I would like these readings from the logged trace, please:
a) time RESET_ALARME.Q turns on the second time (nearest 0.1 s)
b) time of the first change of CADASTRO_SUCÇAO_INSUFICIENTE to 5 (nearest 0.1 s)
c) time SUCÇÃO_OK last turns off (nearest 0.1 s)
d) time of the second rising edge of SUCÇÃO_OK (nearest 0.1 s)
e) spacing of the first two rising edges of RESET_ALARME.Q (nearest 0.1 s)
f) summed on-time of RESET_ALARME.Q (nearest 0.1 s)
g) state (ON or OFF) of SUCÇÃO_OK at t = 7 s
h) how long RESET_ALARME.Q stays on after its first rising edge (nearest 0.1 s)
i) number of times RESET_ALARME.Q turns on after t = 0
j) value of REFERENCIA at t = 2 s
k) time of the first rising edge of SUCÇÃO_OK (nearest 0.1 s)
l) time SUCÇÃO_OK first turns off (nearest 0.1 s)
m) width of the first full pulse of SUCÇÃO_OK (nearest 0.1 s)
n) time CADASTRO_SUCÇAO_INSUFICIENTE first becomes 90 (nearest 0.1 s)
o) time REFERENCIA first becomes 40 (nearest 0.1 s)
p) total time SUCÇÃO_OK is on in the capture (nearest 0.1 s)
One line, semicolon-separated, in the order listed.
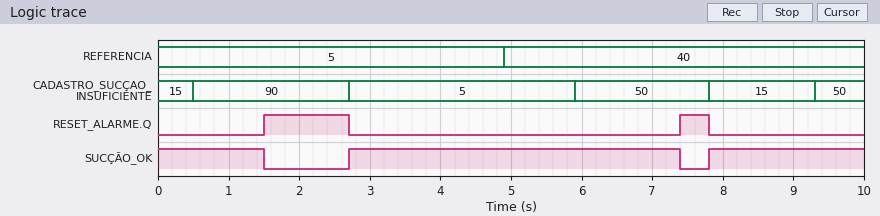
7.4 s; 2.7 s; 7.4 s; 7.8 s; 5.9 s; 1.6 s; ON; 1.2 s; 2; 5; 2.7 s; 1.5 s; 4.7 s; 0.5 s; 4.9 s; 8.4 s
